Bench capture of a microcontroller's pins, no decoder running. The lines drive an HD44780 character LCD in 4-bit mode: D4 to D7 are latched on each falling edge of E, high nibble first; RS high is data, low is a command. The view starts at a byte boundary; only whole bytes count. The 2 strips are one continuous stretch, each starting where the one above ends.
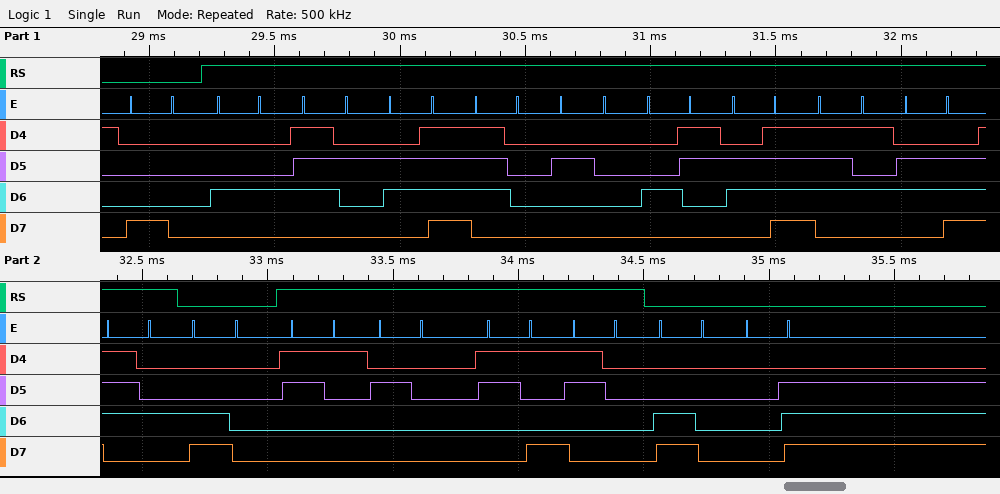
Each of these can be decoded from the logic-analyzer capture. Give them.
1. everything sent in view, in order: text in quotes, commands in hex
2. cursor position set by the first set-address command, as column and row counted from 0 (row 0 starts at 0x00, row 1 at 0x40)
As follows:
0x80 "Drop Count" 0xC0 "1 90" 0xC0 0x0E
column 0, row 0
